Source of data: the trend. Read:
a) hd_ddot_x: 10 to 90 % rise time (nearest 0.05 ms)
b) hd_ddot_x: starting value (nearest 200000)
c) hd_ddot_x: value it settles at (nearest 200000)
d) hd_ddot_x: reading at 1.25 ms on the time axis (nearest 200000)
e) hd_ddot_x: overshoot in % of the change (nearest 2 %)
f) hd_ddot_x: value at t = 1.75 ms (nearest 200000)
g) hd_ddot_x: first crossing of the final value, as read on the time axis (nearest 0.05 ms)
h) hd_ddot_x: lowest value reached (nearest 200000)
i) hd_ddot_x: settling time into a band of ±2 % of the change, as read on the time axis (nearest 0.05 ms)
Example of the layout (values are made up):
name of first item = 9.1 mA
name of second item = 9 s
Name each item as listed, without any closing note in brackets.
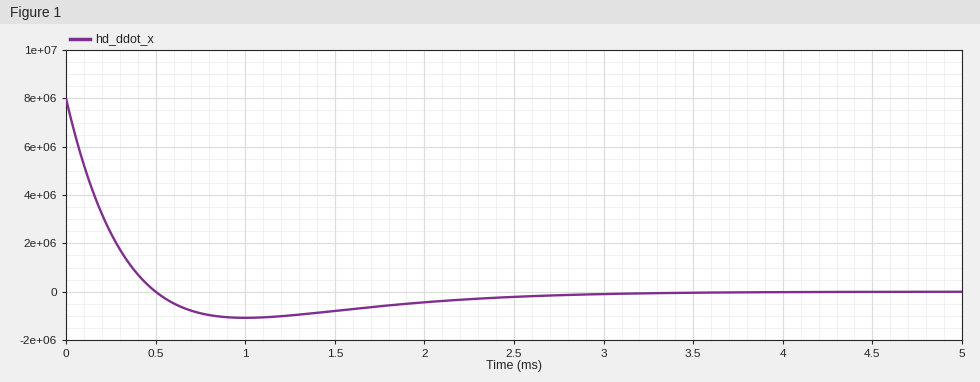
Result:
hd_ddot_x: 10 to 90 % rise time = 0.35 ms
hd_ddot_x: starting value = 8000000
hd_ddot_x: value it settles at = 0
hd_ddot_x: reading at 1.25 ms on the time axis = -1000000
hd_ddot_x: overshoot in % of the change = 14 %
hd_ddot_x: value at t = 1.75 ms = -600000
hd_ddot_x: first crossing of the final value, as read on the time axis = 0.50 ms
hd_ddot_x: lowest value reached = -1000000
hd_ddot_x: settling time into a band of ±2 % of the change, as read on the time axis = 2.70 ms
